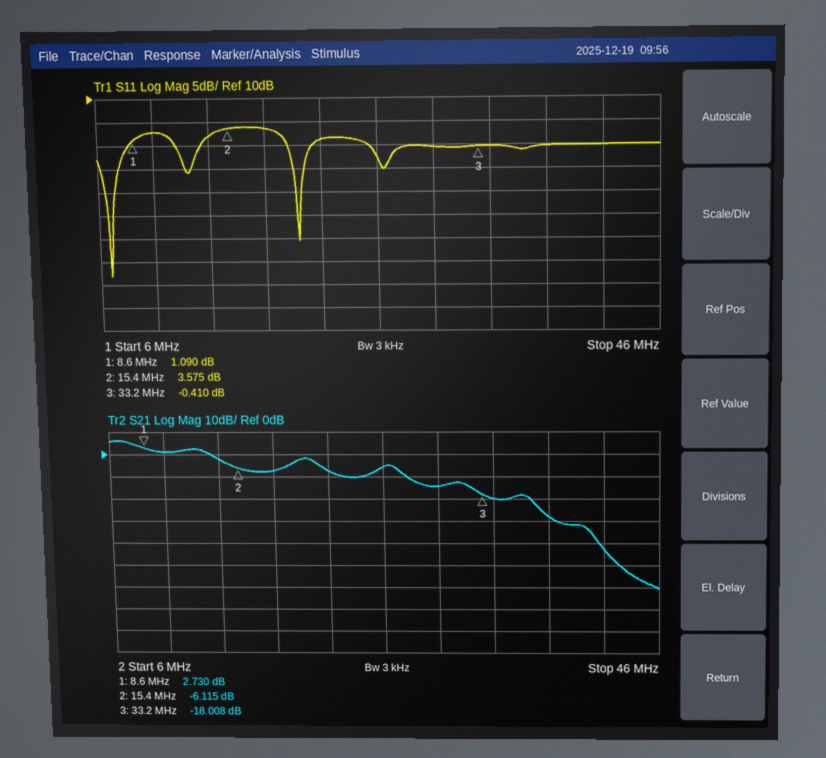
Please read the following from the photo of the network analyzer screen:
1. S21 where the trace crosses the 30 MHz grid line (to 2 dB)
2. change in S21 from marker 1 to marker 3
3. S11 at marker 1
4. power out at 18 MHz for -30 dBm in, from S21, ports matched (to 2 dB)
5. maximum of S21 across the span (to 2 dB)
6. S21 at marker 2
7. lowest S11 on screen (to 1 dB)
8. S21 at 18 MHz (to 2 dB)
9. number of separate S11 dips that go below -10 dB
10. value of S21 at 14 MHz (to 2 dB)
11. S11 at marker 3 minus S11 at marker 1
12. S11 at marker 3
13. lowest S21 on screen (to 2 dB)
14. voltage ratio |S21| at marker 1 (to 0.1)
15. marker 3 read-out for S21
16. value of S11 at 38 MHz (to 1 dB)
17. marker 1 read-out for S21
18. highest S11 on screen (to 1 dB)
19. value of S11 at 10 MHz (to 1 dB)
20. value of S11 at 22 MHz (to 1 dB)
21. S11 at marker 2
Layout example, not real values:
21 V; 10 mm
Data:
-14 dB; -20.738 dB; 1.090 dB; -38 dBm; 6 dB; -6.115 dB; -28 dB; -8 dB; 2; -2 dB; -1.500 dB; -0.410 dB; -60 dB; 1.4; -18.008 dB; 0 dB; 2.730 dB; 4 dB; 3 dB; 1 dB; 3.575 dB
